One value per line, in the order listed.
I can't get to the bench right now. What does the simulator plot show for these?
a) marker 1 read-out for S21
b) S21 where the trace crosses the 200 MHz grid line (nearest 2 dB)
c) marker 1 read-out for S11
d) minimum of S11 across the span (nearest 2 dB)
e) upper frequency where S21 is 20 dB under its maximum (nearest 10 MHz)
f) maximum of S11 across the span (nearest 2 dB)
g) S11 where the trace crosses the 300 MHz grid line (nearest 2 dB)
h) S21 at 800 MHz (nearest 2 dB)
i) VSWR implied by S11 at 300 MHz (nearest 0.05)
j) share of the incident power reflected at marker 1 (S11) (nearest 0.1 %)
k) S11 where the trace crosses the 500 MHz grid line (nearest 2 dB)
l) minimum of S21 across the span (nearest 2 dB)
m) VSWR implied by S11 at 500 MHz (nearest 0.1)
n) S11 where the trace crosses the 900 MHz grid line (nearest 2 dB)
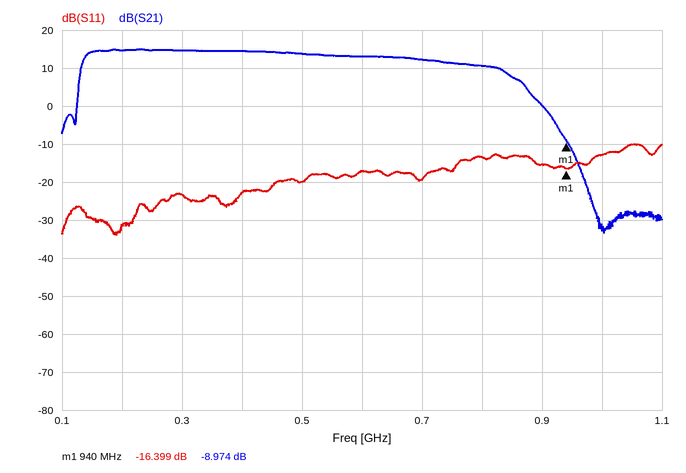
-8.974 dB
14 dB
-16.399 dB
-34 dB
920 MHz
-10 dB
-24 dB
10 dB
1.15
2.3 %
-20 dB
-34 dB
1.2
-16 dB
